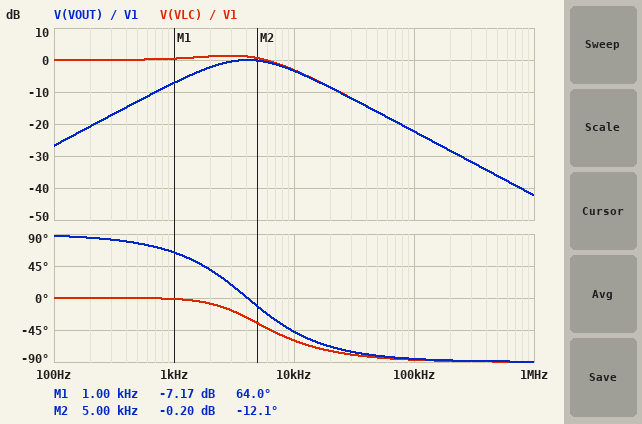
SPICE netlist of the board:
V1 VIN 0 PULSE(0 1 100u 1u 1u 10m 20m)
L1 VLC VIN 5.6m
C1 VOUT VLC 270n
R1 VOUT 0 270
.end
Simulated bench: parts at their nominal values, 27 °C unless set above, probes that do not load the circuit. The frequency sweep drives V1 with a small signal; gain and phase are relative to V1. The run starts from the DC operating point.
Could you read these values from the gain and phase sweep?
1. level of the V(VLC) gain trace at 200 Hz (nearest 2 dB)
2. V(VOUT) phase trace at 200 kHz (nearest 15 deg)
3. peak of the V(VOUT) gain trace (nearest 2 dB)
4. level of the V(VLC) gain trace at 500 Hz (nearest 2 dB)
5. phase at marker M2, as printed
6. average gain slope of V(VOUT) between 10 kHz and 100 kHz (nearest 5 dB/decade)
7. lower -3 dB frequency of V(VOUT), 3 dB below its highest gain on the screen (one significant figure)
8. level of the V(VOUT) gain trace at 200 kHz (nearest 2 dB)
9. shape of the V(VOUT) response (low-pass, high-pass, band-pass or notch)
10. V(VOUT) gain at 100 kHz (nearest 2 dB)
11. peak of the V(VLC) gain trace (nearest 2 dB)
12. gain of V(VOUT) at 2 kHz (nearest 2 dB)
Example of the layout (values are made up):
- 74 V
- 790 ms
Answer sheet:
- 0 dB
- -90 deg
- 0 dB
- 0 dB
- -12.1 deg
- -20 dB/decade
- 2 kHz
- -28 dB
- band-pass
- -22 dB
- 2 dB
- -2 dB
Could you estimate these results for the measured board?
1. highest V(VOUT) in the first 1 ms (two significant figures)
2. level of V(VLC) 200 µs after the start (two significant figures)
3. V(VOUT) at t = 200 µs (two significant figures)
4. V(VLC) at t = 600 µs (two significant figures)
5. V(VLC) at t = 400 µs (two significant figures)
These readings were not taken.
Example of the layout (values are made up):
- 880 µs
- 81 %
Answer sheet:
- 720 mV
- 1.1 V
- 380 mV
- 1.0 V
- 1.0 V
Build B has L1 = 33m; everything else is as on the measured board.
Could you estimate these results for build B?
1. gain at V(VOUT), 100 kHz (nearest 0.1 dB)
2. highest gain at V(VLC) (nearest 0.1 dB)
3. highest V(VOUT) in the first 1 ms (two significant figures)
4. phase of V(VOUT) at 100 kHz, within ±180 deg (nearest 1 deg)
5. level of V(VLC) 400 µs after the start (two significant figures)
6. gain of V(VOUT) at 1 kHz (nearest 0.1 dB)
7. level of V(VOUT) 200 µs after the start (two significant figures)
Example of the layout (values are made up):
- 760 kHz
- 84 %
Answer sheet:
- -37.7 dB
- 4.6 dB
- 470 mV
- -89 deg
- 1.3 V
- -4.8 dB
- 460 mV
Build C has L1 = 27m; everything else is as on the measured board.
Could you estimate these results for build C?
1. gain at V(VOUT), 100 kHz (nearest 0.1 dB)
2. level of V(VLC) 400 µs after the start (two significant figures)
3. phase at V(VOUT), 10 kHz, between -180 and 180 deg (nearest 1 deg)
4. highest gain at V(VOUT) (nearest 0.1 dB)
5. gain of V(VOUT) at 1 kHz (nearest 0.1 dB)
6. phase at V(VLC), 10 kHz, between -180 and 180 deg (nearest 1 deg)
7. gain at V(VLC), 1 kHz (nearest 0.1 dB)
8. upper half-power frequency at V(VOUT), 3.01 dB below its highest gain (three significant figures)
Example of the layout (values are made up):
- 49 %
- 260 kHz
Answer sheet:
- -36.0 dB
- 1.2 V
- -81 deg
- 0 dB
- -5.3 dB
- -93 deg
- 2.3 dB
- 2.82 kHz
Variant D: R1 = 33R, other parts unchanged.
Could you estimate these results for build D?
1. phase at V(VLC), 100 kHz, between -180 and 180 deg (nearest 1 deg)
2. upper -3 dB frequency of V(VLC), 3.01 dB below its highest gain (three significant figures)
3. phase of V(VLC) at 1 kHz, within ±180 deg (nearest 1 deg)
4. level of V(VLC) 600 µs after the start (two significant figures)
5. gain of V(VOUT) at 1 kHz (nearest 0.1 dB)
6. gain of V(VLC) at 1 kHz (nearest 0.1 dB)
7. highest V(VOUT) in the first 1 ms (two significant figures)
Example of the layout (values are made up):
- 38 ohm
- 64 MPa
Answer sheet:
- -100 deg
- 4.49 kHz
- 0 deg
- 780 mV
- -24.5 dB
- 0.5 dB
- 190 mV
